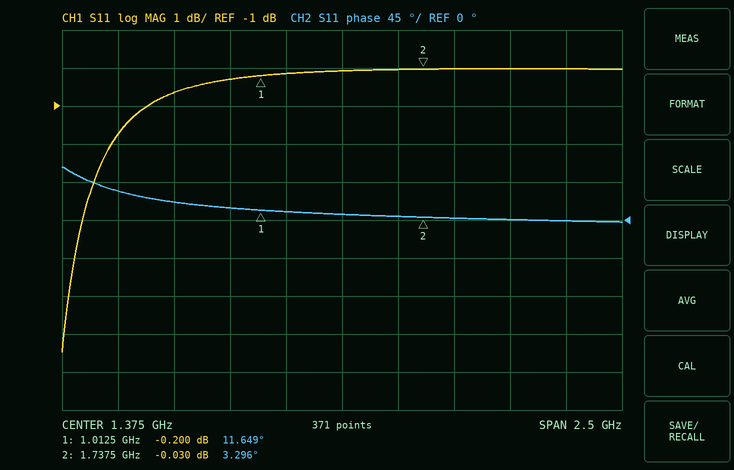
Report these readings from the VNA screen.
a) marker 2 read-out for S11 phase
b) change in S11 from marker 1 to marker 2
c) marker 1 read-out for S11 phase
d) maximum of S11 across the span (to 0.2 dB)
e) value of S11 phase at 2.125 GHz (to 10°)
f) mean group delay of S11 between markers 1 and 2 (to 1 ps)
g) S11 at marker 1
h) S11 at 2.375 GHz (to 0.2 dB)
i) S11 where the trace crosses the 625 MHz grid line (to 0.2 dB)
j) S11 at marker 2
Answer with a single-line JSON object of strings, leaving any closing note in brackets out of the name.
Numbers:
{"marker 2 read-out for S11 phase": "3.296°", "change in S11 from marker 1 to marker 2": "0.170 dB", "marker 1 read-out for S11 phase": "11.649°", "maximum of S11 across the span": "0.0 dB", "value of S11 phase at 2.125 GHz": "0°", "mean group delay of S11 between markers 1 and 2": "32 ps", "S11 at marker 1": "-0.200 dB", "S11 at 2.375 GHz": "0.0 dB", "S11 where the trace crosses the 625 MHz grid line": "-0.6 dB", "S11 at marker 2": "-0.030 dB"}
